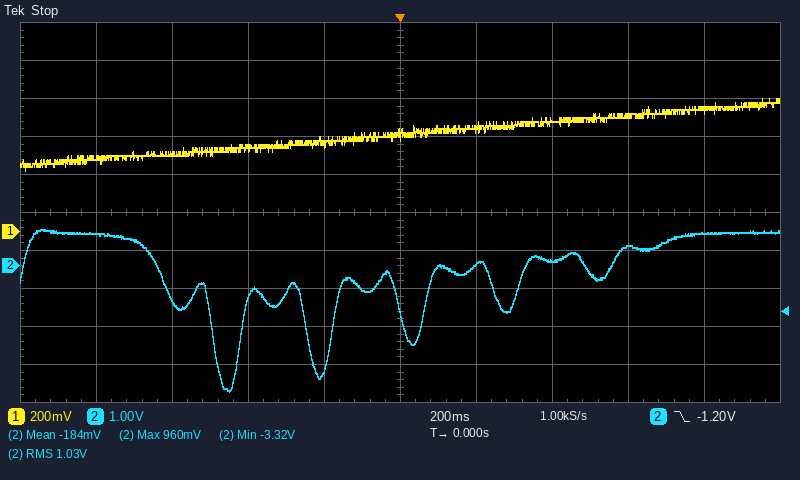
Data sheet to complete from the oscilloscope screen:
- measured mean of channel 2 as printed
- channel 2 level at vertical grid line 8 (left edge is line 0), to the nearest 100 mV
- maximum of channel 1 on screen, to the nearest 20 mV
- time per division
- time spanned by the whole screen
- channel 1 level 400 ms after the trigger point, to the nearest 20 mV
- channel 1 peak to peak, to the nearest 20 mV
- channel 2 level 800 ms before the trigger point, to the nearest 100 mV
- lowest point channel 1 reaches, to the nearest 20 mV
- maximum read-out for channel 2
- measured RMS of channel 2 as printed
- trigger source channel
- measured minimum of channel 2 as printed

-184 mV
500 mV
700 mV
200 ms
2 s
580 mV
380 mV
800 mV
320 mV
960 mV
1.03 V
channel 2
-3.32 V
